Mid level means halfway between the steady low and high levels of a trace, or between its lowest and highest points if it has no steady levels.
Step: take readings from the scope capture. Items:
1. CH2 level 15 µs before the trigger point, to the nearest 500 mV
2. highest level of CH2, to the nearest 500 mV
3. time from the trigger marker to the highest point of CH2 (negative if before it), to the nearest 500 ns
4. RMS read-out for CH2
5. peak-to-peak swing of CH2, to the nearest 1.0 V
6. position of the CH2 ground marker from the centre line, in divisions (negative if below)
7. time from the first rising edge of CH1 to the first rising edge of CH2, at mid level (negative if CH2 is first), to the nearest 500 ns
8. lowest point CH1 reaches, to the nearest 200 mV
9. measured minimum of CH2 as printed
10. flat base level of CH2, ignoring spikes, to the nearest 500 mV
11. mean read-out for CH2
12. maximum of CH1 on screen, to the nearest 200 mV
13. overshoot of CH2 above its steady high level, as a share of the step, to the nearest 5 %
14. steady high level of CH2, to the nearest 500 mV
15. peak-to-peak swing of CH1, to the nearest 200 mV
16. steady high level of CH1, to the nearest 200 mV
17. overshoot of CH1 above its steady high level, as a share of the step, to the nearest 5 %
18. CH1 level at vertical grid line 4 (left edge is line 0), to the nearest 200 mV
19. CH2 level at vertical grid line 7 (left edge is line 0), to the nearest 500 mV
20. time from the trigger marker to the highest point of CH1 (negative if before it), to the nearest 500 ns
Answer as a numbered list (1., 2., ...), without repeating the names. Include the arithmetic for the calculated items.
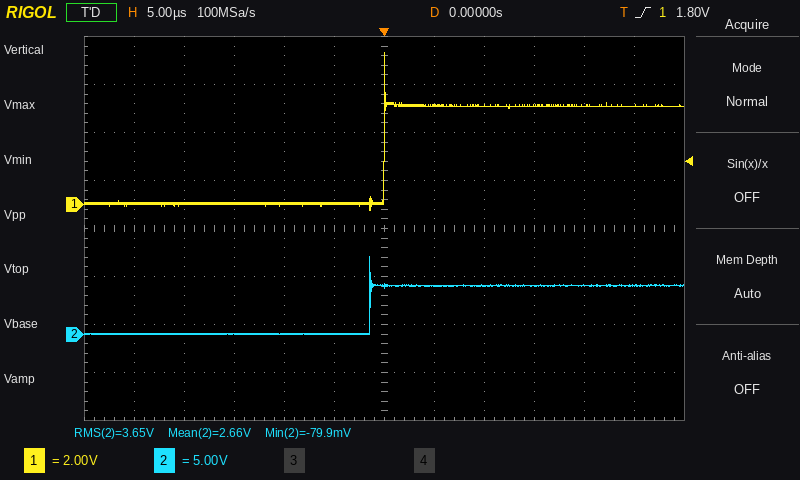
1. 0.0 V
2. 8.0 V
3. -1.5 µs
4. 3.65 V
5. 8.0 V
6. -2.2 div
7. -1.5 µs
8. -200 mV
9. -79.9 mV
10. 0.0 V
11. 2.66 V
12. 6.4 V
13. 60 %
14. 5.0 V
15. 6.4 V − (-200 mV) = 6.6 V
16. 4.0 V
17. 55 %
18. 0.0 V
19. 5.0 V
20. 0.0 µs
